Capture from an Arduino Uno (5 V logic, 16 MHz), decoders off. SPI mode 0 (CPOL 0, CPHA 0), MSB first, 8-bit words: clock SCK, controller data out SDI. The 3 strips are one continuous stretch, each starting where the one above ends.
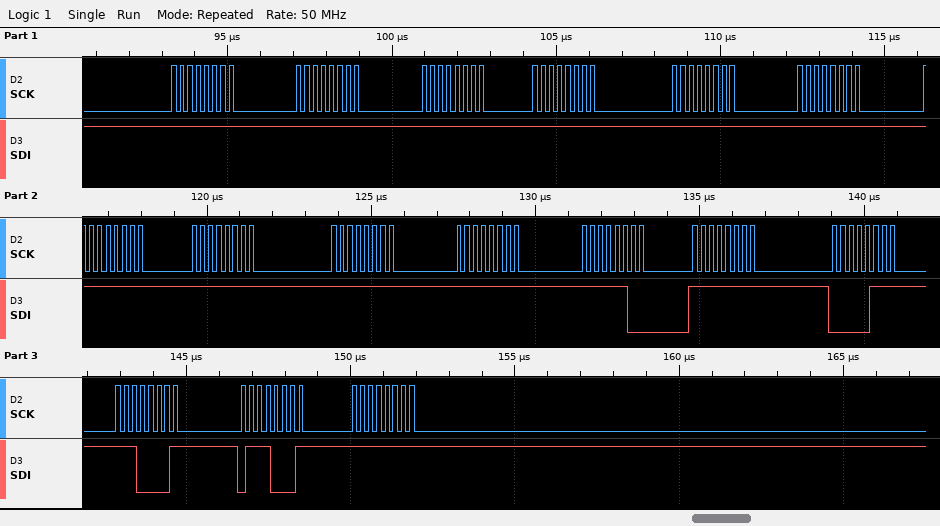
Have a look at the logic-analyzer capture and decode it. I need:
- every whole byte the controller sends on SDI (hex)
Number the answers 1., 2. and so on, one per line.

1. 0xFF 0xFF 0xFF 0xFF 0xFF 0xFF 0xFF 0xFF 0xFF 0xFF 0xFC 0xFF 0x07 0xE1 0x71 0xFF
